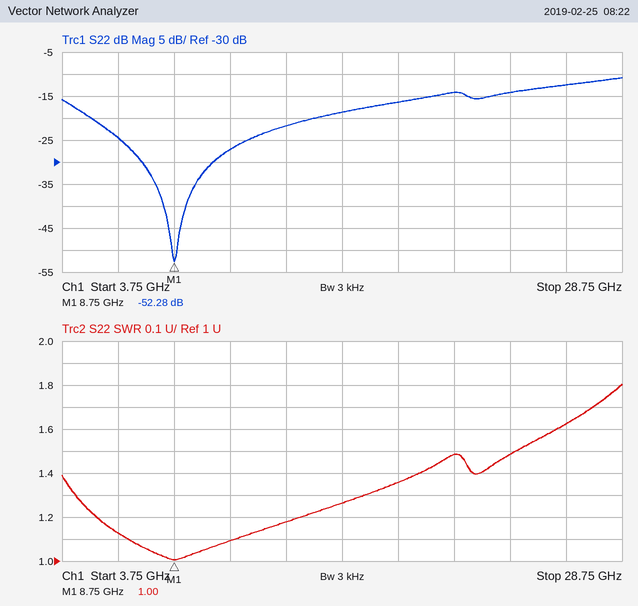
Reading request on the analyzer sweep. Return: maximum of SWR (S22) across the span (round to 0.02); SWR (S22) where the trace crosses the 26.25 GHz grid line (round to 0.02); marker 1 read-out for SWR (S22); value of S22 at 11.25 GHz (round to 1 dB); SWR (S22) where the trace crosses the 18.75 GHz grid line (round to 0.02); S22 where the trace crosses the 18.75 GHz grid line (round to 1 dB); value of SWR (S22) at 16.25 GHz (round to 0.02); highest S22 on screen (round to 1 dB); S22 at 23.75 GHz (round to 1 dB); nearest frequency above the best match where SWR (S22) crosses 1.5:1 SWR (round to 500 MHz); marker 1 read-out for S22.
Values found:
1.80
1.62
1.00
-27 dB
1.36
-16 dB
1.26
-11 dB
-14 dB
24.0 GHz
-52.28 dB
